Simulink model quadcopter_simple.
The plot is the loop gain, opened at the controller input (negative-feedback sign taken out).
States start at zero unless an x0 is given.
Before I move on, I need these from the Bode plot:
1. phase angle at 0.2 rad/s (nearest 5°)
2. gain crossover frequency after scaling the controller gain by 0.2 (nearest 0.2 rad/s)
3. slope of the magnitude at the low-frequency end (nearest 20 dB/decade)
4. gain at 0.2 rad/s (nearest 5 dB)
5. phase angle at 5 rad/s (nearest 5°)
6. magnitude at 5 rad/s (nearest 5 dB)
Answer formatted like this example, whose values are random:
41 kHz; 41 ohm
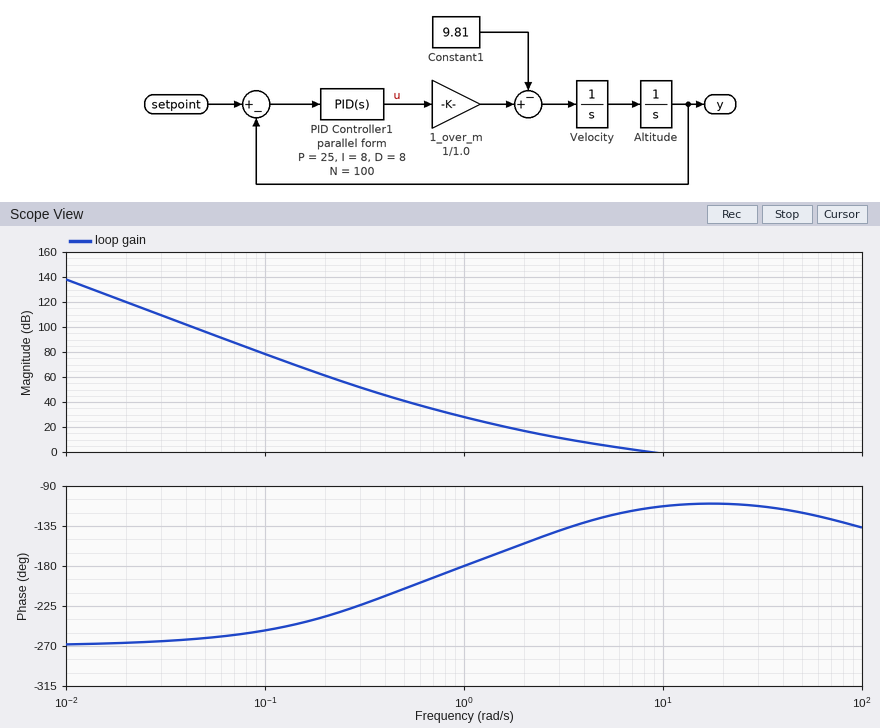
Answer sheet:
-235°; 2.4 rad/s; -60 dB/decade; 60 dB; -125°; 5 dB
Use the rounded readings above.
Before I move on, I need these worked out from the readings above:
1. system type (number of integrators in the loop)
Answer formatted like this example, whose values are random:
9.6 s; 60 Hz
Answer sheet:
3
